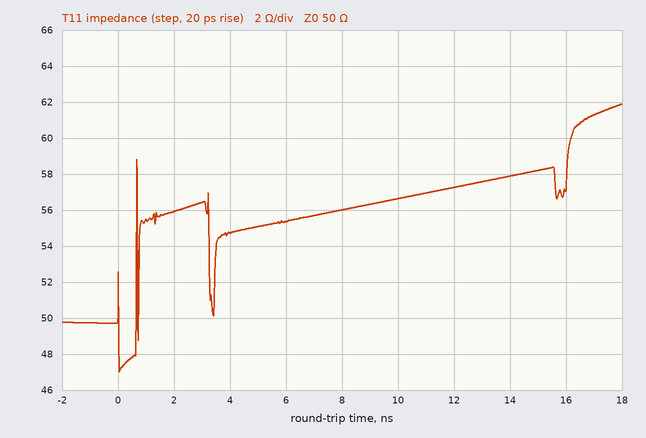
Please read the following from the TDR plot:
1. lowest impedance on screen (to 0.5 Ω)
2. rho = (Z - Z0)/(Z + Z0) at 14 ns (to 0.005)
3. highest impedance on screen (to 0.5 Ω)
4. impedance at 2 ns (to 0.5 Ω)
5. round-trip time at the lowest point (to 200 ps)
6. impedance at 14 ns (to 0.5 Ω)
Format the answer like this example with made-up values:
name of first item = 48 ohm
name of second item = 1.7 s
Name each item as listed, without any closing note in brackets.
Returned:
lowest impedance on screen = 47.0 Ω
rho = (Z - Z0)/(Z + Z0) at 14 ns = +0.075
highest impedance on screen = 62.0 Ω
impedance at 2 ns = 56.0 Ω
round-trip time at the lowest point = 0.0 ns
impedance at 14 ns = 58.0 Ω
